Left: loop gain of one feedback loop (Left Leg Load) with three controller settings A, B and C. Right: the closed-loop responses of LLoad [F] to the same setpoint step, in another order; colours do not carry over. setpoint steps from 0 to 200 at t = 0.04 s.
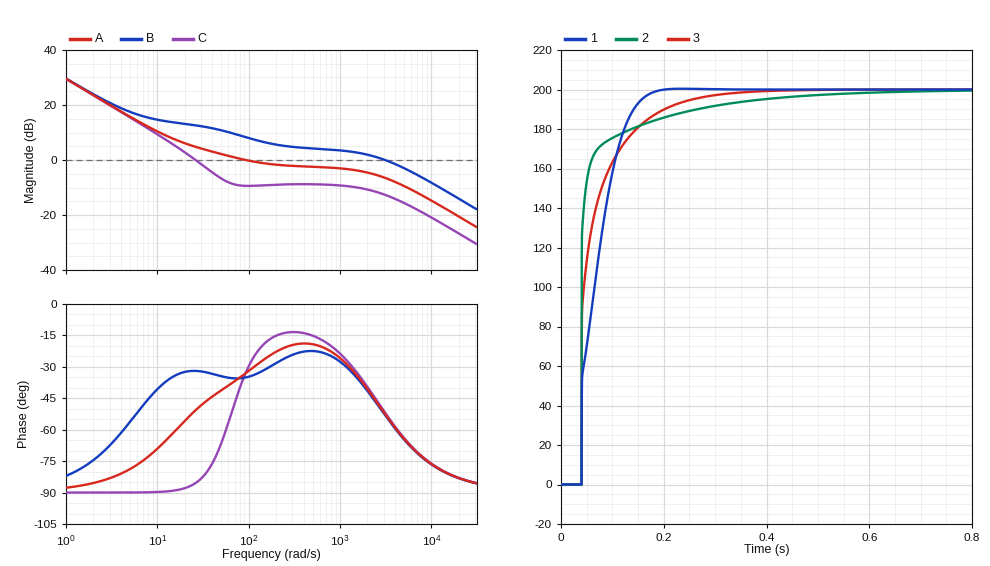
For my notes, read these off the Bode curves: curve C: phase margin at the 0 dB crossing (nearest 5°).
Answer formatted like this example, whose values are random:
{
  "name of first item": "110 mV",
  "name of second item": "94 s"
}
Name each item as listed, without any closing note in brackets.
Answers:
{
  "curve C: phase margin at the 0 dB crossing": "95°"
}
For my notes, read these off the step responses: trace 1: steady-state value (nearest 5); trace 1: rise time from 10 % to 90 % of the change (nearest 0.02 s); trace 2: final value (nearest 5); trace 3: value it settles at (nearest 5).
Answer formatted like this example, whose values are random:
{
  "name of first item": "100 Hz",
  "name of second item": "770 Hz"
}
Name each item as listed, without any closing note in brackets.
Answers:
{
  "trace 1: steady-state value": "200",
  "trace 1: rise time from 10 % to 90 % of the change": "0.08 s",
  "trace 2: final value": "200",
  "trace 3: value it settles at": "200"
}
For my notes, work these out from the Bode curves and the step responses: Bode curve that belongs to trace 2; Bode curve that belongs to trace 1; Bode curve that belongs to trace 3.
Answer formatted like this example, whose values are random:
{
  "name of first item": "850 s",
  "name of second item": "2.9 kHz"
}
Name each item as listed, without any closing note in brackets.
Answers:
{
  "Bode curve that belongs to trace 2": "B",
  "Bode curve that belongs to trace 1": "C",
  "Bode curve that belongs to trace 3": "A"
}
